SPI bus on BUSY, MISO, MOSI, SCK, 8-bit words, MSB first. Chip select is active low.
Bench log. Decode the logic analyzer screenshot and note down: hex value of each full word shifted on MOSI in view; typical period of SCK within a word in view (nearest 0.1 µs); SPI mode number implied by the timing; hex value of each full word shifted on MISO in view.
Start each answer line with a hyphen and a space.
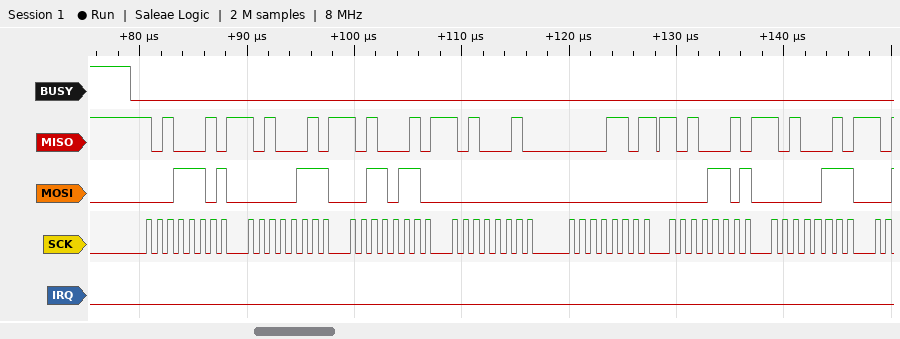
- 1D, 07, 36, 00, 00, 0D, 07
- 1 µs
- 0
- A2, A2, A2, A2, 0D, A2, A2
